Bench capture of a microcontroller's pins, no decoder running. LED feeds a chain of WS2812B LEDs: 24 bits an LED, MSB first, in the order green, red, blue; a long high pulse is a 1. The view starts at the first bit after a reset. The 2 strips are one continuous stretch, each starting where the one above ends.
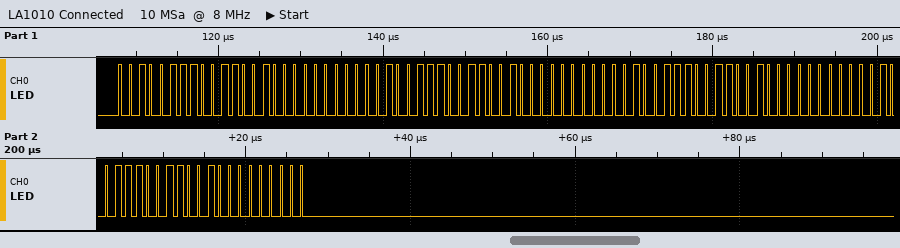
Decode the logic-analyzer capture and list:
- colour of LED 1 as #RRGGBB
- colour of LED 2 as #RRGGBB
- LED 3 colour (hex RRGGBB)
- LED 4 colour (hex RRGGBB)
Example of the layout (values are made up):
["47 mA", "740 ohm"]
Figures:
["#322700", "#322700", "#322700", "#322700"]
